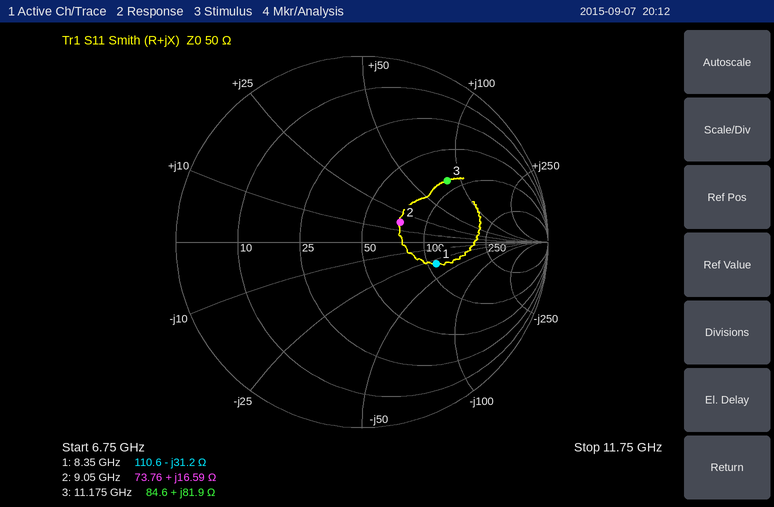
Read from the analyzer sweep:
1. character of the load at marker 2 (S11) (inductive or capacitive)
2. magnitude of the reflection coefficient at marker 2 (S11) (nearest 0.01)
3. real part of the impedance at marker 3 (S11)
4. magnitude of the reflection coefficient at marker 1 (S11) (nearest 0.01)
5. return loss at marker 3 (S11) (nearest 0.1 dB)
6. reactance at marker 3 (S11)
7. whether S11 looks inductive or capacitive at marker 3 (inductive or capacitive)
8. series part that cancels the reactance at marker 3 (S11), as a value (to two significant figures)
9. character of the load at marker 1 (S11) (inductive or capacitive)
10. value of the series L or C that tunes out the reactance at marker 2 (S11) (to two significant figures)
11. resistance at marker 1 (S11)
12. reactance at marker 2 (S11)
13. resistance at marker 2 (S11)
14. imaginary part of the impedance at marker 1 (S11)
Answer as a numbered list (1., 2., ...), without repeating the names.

1. inductive
2. 0.23
3. 84.6 Ω
4. 0.42
5. 5.0 dB
6. +81.9 Ω
7. inductive
8. 170 fF
9. capacitive
10. 1.1 pF
11. 110.6 Ω
12. +16.59 Ω
13. 73.76 Ω
14. -31.2 Ω
